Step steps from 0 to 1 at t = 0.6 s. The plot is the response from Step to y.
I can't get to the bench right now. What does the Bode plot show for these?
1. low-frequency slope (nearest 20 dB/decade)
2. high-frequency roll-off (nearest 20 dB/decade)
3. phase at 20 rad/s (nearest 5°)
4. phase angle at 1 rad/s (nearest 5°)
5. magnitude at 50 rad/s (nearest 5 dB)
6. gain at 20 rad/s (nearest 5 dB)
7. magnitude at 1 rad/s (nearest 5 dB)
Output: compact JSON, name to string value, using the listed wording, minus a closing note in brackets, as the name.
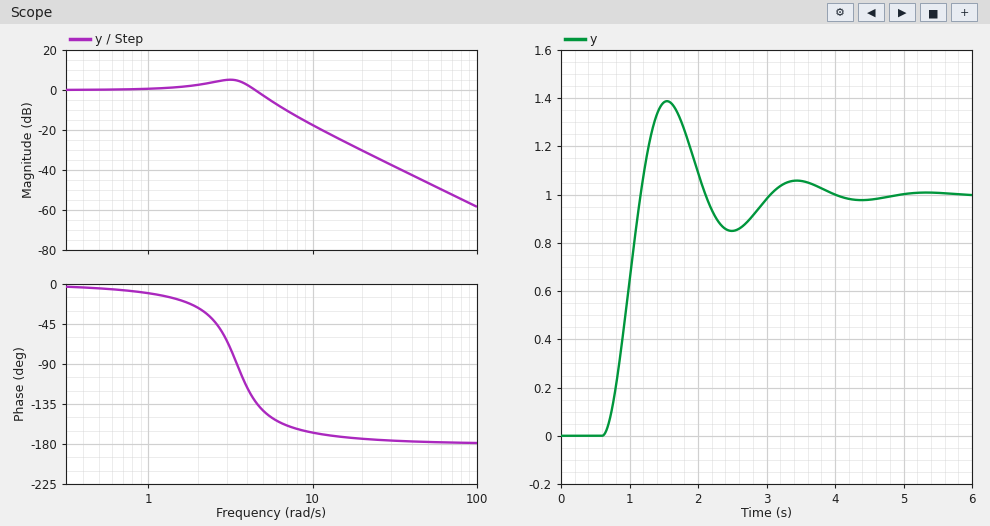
{"low-frequency slope": "0 dB/decade", "high-frequency roll-off": "-40 dB/decade", "phase at 20 rad/s": "-175°", "phase angle at 1 rad/s": "-10°", "magnitude at 50 rad/s": "-45 dB", "gain at 20 rad/s": "-30 dB", "magnitude at 1 rad/s": "0 dB"}
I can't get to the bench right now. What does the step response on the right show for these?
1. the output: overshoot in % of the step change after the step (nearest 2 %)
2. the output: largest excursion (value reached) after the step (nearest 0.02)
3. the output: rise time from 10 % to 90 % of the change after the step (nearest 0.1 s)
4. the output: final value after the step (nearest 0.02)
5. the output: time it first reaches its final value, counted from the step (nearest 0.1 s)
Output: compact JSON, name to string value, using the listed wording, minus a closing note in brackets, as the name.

{"the output: overshoot in % of the step change after the step": "38 %", "the output: largest excursion (value reached) after the step": "1.38", "the output: rise time from 10 % to 90 % of the change after the step": "0.4 s", "the output: final value after the step": "1.00", "the output: time it first reaches its final value, counted from the step": "0.6 s"}
